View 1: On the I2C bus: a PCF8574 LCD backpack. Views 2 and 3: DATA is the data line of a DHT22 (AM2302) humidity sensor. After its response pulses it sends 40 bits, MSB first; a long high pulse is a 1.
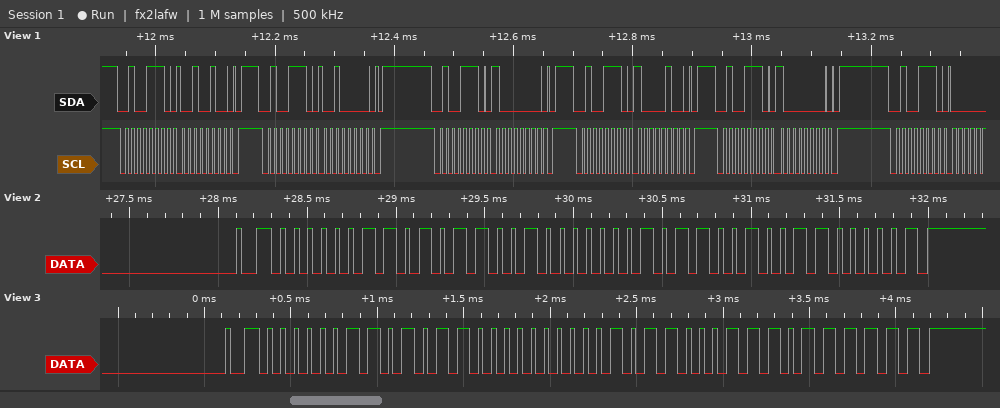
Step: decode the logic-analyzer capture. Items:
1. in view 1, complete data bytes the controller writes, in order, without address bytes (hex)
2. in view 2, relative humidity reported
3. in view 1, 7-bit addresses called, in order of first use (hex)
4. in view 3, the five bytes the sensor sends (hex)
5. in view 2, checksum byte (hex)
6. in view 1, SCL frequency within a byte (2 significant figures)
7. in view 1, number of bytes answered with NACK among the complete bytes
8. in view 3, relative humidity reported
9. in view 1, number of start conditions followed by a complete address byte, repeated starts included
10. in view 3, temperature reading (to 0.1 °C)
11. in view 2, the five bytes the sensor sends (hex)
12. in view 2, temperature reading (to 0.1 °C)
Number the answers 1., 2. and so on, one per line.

1. 24 20 80 84 80
2. 85.7 %
3. 0x27
4. 03 58 01 63 BF
5. 0xC1
6. 100 kHz
7. 0
8. 85.6 %
9. 6
10. 35.5 °C
11. 03 59 01 64 C1
12. 35.6 °C
